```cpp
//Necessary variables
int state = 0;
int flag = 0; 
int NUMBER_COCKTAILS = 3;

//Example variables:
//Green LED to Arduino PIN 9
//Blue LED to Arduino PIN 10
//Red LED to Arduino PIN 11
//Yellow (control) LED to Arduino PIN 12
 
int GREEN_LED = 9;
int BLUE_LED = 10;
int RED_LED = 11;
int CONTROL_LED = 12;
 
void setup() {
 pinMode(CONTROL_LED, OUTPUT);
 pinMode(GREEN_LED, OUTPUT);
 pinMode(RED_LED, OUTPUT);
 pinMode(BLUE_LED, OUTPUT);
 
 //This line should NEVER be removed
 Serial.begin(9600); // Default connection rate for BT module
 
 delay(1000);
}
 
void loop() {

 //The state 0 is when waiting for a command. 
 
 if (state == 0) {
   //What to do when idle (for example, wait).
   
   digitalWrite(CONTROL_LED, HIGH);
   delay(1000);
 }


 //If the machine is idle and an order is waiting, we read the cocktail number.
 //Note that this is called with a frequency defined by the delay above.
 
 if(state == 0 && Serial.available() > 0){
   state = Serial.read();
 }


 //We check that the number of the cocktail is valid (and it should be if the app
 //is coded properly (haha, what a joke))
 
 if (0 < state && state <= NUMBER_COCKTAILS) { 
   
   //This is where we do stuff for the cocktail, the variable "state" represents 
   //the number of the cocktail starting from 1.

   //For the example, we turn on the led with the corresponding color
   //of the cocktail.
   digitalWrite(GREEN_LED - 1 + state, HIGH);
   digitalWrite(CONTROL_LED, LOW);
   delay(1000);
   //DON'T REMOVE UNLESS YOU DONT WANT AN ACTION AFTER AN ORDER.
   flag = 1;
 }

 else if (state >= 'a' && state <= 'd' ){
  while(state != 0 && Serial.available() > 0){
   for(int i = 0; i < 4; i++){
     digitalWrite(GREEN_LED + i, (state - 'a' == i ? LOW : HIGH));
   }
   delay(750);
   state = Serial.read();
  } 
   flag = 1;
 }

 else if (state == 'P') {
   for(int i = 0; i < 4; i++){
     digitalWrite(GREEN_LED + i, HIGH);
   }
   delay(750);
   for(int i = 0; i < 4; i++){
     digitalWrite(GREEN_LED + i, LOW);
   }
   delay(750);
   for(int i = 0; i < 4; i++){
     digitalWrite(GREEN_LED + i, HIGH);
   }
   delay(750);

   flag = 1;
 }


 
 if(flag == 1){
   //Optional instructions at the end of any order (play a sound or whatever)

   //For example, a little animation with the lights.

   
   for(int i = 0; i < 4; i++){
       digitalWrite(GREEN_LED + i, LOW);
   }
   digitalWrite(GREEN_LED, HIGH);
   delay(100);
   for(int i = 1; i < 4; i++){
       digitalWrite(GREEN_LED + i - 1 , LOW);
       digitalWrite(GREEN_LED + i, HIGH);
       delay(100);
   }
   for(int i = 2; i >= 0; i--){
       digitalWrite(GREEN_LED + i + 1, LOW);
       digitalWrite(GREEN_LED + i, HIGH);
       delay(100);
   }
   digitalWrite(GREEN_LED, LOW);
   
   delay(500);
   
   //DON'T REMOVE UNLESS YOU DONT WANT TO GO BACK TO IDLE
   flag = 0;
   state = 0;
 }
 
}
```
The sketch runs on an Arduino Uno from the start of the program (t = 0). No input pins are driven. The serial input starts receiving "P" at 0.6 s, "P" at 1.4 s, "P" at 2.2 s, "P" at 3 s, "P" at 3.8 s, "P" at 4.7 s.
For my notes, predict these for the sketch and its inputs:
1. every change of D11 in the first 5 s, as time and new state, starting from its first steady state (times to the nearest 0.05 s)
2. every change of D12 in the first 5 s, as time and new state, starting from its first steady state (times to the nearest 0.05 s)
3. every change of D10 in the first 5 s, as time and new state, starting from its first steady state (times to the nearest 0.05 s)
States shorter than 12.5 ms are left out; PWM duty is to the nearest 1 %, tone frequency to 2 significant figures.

0 s low; 2 s high; 2.75 s low; 3.5 s high; 4.25 s low; 4.45 s high; 4.55 s low; 4.65 s high; 4.75 s low
0 s low; 1 s high; 2.75 s low; 3.5 s high; 4.25 s low; 4.55 s high; 4.65 s low
0 s low; 2 s high; 2.75 s low; 3.5 s high; 4.25 s low; 4.35 s high; 4.45 s low; 4.75 s high; 4.85 s low
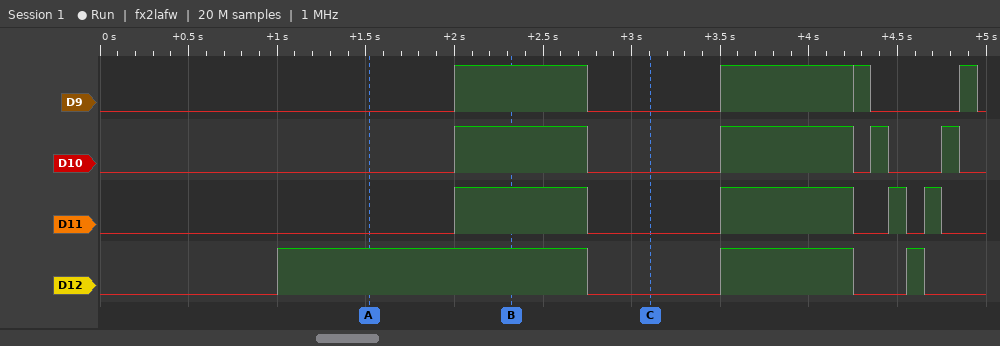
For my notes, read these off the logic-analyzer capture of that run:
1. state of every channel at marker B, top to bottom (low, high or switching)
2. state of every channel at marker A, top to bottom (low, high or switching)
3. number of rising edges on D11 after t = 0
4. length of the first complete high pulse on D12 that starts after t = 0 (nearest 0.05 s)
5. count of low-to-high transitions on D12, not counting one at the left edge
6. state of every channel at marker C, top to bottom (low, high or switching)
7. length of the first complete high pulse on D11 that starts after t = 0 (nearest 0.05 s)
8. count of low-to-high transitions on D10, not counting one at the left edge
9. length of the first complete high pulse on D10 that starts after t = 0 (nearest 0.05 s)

D9 high, D10 high, D11 high, D12 high
D9 low, D10 low, D11 low, D12 high
4
1.75 s
3
D9 low, D10 low, D11 low, D12 low
0.75 s
4
0.75 s
